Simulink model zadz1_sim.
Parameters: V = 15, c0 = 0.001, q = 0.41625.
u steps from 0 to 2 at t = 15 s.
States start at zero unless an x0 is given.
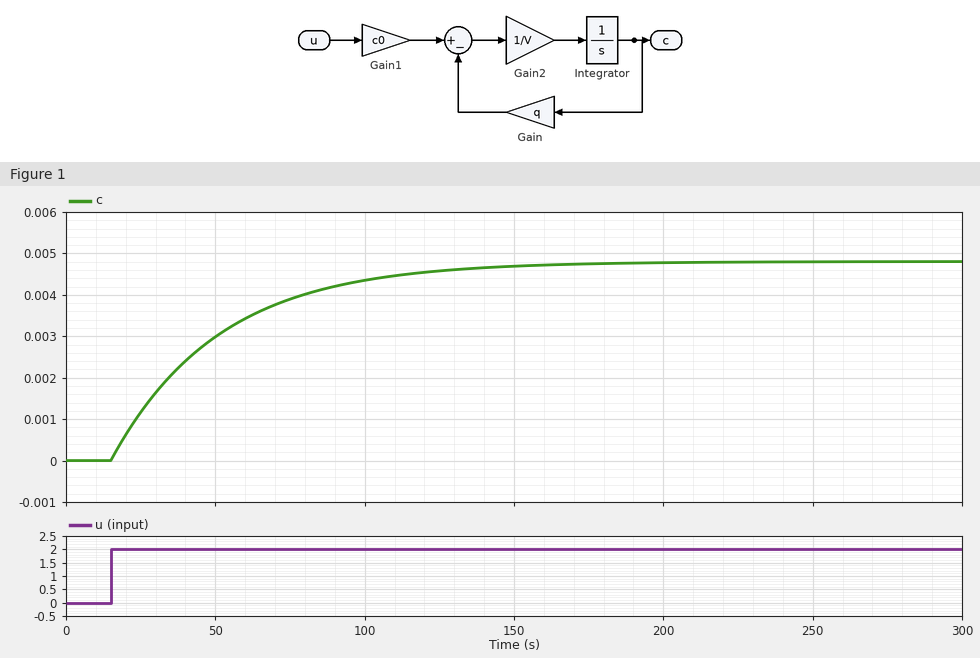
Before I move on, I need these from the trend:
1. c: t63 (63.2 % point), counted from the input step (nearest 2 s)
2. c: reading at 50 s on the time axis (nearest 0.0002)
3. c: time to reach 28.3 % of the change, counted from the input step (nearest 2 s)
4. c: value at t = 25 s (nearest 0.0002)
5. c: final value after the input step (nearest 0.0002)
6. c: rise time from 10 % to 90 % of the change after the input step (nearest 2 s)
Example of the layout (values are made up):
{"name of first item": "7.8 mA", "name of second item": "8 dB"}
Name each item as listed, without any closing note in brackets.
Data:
{"c: t63 (63.2 % point), counted from the input step": "36 s", "c: reading at 50 s on the time axis": "0.0030", "c: time to reach 28.3 % of the change, counted from the input step": "12 s", "c: value at t = 25 s": "0.0012", "c: final value after the input step": "0.0048", "c: rise time from 10 % to 90 % of the change after the input step": "80 s"}
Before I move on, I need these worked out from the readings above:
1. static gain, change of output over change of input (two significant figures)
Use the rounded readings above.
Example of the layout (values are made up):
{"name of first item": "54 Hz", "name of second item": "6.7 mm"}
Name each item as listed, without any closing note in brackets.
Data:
{"static gain, change of output over change of input": "0.0024"}
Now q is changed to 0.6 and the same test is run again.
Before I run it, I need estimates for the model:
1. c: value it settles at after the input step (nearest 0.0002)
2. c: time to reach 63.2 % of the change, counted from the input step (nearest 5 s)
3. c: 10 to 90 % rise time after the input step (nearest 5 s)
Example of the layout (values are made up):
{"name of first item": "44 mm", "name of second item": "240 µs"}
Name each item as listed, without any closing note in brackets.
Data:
{"c: value it settles at after the input step": "0.0034", "c: time to reach 63.2 % of the change, counted from the input step": "25 s", "c: 10 to 90 % rise time after the input step": "55 s"}
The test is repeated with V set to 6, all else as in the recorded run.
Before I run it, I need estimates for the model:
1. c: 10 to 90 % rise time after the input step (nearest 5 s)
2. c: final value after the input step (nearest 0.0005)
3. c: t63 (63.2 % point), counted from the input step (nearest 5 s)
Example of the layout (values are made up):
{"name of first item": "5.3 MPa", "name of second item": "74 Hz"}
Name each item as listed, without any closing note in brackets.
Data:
{"c: 10 to 90 % rise time after the input step": "30 s", "c: final value after the input step": "0.0050", "c: t63 (63.2 % point), counted from the input step": "15 s"}
